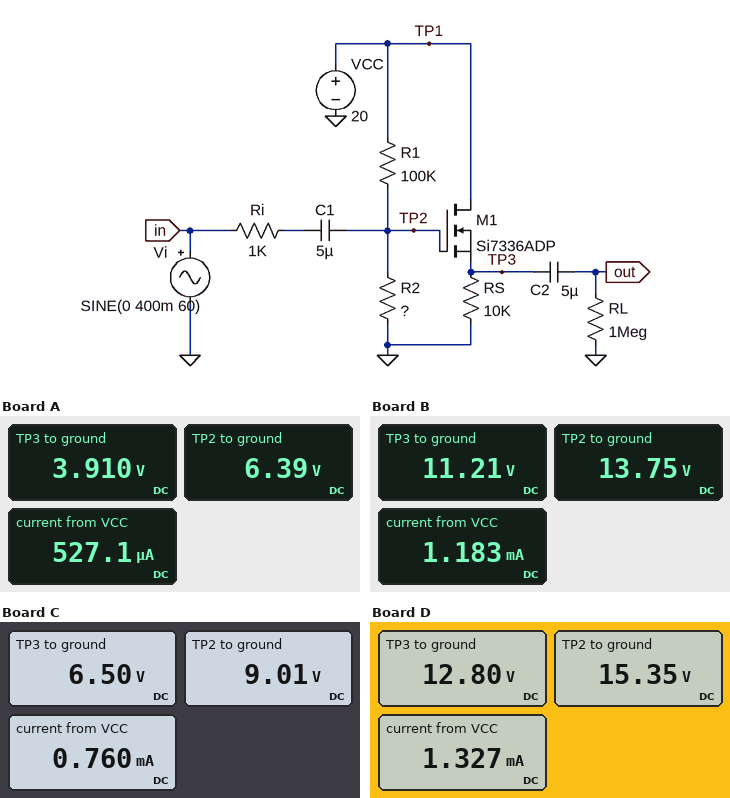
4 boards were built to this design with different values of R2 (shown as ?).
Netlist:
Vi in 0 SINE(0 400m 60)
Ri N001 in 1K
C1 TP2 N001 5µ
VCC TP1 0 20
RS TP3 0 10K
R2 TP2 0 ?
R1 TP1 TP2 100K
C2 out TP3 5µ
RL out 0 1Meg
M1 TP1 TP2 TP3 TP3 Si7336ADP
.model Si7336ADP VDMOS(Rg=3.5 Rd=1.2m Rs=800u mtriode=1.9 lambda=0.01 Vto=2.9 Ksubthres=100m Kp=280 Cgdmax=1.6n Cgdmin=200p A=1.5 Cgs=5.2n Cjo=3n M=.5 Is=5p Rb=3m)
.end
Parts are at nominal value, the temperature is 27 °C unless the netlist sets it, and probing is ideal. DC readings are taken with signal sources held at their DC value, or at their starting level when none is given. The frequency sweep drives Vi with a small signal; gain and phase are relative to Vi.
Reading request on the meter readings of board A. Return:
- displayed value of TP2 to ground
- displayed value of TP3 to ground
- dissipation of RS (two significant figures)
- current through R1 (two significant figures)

6.39 V
3.910 V
1.5 mW
140 µA
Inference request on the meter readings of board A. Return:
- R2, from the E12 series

47 kΩ
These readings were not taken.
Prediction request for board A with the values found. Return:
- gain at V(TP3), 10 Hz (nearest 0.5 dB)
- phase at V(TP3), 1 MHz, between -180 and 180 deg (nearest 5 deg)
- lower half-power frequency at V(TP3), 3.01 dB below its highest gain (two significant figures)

-0.5 dB
-85 deg
1.2 Hz
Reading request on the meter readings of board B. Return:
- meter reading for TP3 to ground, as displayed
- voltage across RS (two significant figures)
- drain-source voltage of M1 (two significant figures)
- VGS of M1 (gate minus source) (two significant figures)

11.21 V
11 V
8.8 V
2.5 V
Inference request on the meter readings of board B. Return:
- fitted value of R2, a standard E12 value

220 kΩ
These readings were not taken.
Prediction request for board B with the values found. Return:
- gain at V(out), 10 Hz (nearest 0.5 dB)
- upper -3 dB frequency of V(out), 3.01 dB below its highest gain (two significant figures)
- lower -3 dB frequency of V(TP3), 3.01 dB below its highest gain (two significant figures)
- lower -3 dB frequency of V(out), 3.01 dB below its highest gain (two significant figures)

0 dB
370 kHz
660 mHz
660 mHz
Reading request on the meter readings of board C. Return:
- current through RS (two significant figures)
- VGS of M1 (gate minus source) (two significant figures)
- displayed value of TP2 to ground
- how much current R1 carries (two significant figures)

650 µA
2.5 V
9.01 V
110 µA
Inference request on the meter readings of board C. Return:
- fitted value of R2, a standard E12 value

82 kΩ
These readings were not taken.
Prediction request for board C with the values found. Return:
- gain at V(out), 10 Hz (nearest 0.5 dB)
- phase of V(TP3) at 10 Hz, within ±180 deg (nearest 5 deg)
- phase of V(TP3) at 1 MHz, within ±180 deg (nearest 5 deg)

-0.5 dB
5 deg
-95 deg
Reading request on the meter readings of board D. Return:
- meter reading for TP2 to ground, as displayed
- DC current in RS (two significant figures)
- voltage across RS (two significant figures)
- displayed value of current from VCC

15.35 V
1.3 mA
13 V
1.327 mA
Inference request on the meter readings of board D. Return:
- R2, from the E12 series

330 kΩ
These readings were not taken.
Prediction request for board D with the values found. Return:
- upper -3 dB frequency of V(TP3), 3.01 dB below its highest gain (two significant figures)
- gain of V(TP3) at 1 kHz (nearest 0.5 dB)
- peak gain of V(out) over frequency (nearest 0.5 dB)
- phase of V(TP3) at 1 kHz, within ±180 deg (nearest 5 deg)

380 kHz
0 dB
1.0 dB
0 deg
